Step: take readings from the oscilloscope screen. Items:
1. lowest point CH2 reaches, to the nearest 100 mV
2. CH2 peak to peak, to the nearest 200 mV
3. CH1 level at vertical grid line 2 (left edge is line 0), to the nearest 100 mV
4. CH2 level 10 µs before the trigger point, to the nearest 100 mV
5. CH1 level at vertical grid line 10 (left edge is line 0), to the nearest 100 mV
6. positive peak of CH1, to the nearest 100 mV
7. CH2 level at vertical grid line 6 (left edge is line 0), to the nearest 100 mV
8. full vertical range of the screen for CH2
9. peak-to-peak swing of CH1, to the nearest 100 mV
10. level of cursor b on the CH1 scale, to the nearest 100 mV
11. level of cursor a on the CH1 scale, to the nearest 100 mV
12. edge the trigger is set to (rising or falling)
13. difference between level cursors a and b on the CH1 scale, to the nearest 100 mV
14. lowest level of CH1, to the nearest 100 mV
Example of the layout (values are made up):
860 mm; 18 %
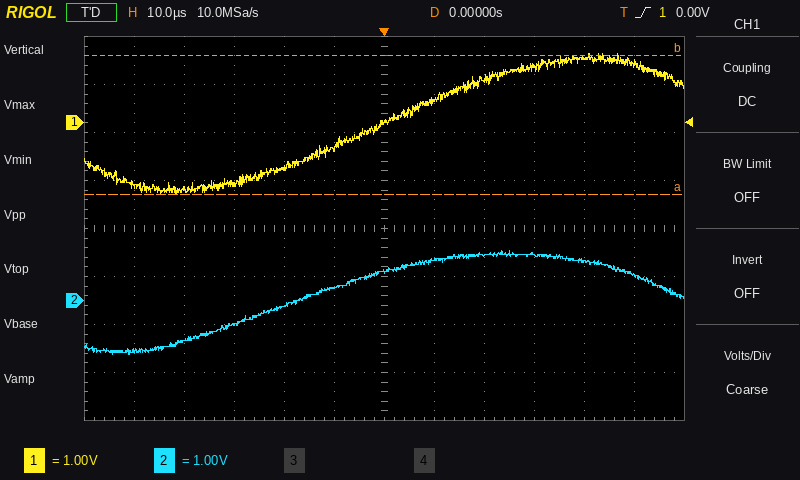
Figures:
-1.1 V; 2.2 V; -1.4 V; 300 mV; 1.4 V; 1.4 V; 600 mV; 8 V; 2.9 V; 1.4 V; -1.5 V; rising; 2.9 V; -1.5 V
